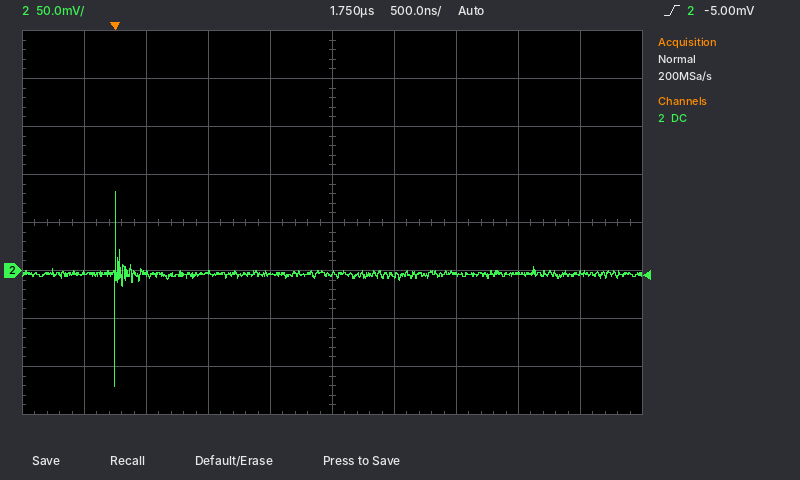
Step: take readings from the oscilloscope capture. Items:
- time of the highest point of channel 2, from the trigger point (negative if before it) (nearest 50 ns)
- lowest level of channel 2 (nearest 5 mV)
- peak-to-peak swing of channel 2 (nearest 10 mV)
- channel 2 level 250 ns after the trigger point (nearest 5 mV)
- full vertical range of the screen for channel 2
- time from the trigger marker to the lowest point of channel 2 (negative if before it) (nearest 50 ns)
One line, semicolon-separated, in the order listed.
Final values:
0 ns; -120 mV; 200 mV; -5 mV; 400 mV; 0 ns
